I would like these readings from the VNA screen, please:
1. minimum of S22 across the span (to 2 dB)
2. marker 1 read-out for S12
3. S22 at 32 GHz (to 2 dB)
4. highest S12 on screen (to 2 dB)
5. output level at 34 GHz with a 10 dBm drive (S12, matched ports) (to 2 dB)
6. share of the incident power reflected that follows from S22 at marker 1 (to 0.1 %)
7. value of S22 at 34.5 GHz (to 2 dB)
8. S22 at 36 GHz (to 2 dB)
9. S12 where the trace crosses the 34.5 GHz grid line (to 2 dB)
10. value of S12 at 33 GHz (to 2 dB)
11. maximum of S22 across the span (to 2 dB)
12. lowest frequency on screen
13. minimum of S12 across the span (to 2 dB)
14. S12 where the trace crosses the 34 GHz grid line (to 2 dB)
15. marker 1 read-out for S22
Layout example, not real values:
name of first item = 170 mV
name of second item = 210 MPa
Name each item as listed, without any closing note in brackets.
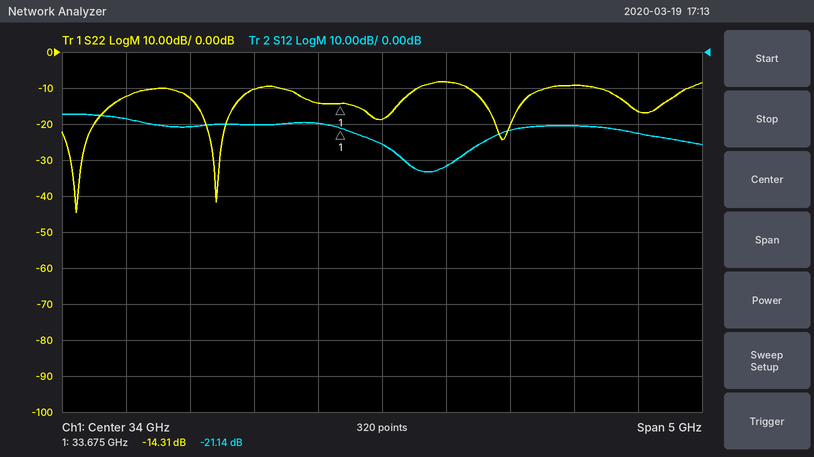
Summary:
minimum of S22 across the span = -44 dB
marker 1 read-out for S12 = -21.14 dB
S22 at 32 GHz = -12 dB
highest S12 on screen = -18 dB
output level at 34 GHz with a 10 dBm drive (S12, matched ports) = -16 dBm
share of the incident power reflected that follows from S22 at marker 1 = 3.7 %
value of S22 at 34.5 GHz = -8 dB
S22 at 36 GHz = -16 dB
S12 where the trace crosses the 34.5 GHz grid line = -32 dB
value of S12 at 33 GHz = -20 dB
maximum of S22 across the span = -8 dB
lowest frequency on screen = 31.5 GHz
minimum of S12 across the span = -34 dB
S12 where the trace crosses the 34 GHz grid line = -26 dB
marker 1 read-out for S22 = -14.31 dB
